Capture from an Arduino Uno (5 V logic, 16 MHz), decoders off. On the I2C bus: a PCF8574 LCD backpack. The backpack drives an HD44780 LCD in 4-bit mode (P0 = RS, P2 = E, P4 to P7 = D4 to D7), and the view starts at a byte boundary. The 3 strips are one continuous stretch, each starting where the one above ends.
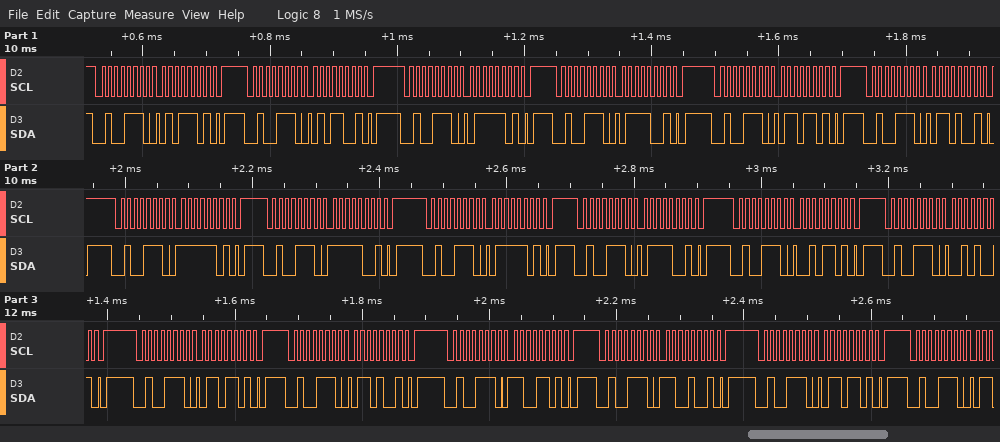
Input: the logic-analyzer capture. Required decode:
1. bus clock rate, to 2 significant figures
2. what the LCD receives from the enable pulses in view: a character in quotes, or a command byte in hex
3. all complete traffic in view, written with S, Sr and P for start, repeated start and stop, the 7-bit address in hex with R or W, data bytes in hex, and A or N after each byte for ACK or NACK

100 kHz
'W' 'o' 'r' 'l'
S 27W A 5D A P S 27W A 59 A P S 27W A 7D A P S 27W A 79 A P S 27W A 6D A P S 27W A 69 A P S 27W A FD A P S 27W A F9 A P S 27W A 7D A P S 27W A 79 A P S 27W A 2D A P S 27W A 29 A P S 27W A 6D A P S 27W A 69 A P S 27W A CD A P S 27W A C9 A P S 27W A 6D A P S 27W A
